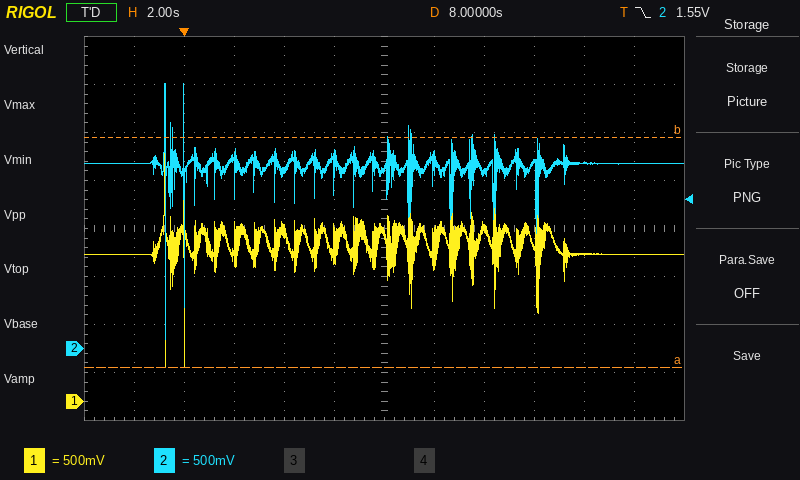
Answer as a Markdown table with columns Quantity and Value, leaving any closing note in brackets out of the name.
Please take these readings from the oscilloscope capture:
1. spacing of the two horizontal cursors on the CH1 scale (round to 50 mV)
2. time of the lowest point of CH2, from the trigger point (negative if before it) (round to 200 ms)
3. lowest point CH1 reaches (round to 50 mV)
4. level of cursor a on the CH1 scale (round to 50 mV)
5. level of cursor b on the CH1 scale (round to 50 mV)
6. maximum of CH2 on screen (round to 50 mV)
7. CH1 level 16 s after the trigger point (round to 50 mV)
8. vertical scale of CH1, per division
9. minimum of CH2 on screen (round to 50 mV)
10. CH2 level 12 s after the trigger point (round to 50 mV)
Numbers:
| Quantity | Value |
|---|---|
| spacing of the two horizontal cursors on the CH1 scale | 2.40 V |
| time of the lowest point of CH2, from the trigger point (negative if before it) | -800 ms |
| lowest point CH1 reaches | 350 mV |
| level of cursor a on the CH1 scale | 350 mV |
| level of cursor b on the CH1 scale | 2.75 V |
| maximum of CH2 on screen | 2.75 V |
| CH1 level 16 s after the trigger point | 1.55 V |
| vertical scale of CH1, per division | 500 mV |
| minimum of CH2 on screen | 100 mV |
| CH2 level 12 s after the trigger point | 1.85 V |
